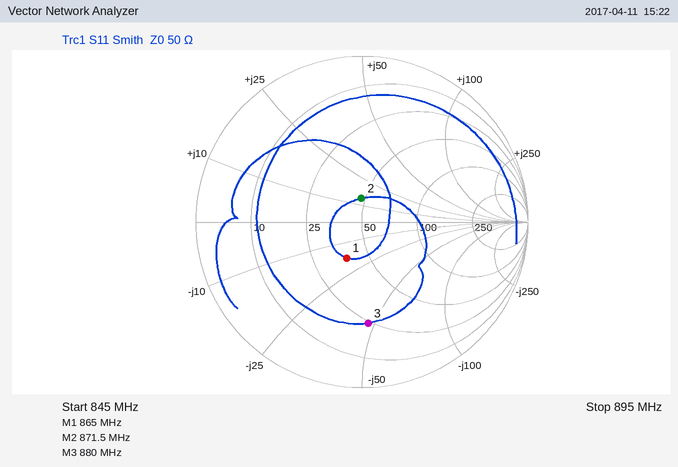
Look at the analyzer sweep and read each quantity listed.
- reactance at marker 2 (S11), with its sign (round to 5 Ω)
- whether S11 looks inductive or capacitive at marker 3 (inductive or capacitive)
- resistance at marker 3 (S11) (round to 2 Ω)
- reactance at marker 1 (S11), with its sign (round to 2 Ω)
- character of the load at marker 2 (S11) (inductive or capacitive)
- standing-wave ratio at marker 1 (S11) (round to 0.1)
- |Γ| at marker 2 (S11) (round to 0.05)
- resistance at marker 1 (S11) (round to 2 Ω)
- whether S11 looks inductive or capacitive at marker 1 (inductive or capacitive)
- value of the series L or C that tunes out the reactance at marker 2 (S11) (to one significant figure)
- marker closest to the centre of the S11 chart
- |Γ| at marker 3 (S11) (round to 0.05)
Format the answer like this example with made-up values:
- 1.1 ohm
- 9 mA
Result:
- +15 Ω
- capacitive
- 24 Ω
- -18 Ω
- inductive
- 1.6
- 0.15
- 38 Ω
- capacitive
- 10 pF
- marker 2
- 0.60
